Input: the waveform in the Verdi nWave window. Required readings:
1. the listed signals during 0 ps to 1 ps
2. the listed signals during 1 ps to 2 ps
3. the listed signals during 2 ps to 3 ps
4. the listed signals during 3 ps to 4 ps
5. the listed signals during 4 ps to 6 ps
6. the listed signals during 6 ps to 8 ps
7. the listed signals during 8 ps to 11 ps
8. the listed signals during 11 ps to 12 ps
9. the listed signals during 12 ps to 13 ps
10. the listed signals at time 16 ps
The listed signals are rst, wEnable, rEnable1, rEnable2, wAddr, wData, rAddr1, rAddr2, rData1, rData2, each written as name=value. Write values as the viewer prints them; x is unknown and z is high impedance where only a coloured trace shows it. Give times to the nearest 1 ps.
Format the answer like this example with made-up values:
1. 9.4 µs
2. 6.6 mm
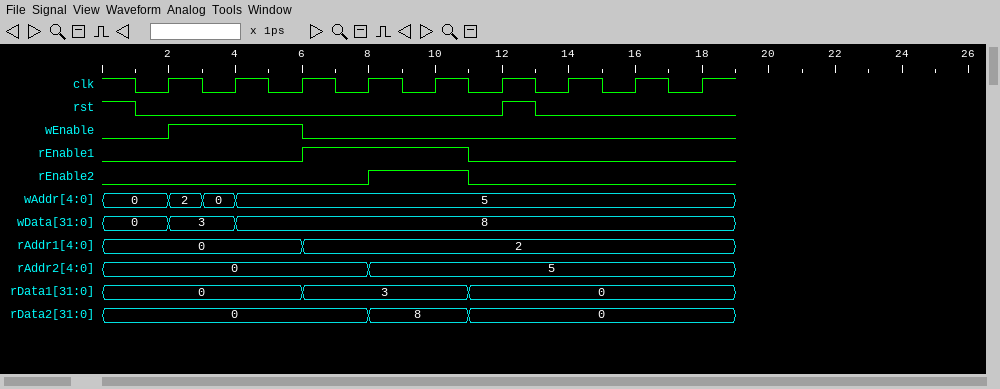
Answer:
1. rst=1, wEnable=0, rEnable1=0, rEnable2=0, wAddr=0, wData=0, rAddr1=0, rAddr2=0, rData1=0, rData2=0
2. rst=0, wEnable=0, rEnable1=0, rEnable2=0, wAddr=0, wData=0, rAddr1=0, rAddr2=0, rData1=0, rData2=0
3. rst=0, wEnable=1, rEnable1=0, rEnable2=0, wAddr=2, wData=3, rAddr1=0, rAddr2=0, rData1=0, rData2=0
4. rst=0, wEnable=1, rEnable1=0, rEnable2=0, wAddr=0, wData=3, rAddr1=0, rAddr2=0, rData1=0, rData2=0
5. rst=0, wEnable=1, rEnable1=0, rEnable2=0, wAddr=5, wData=8, rAddr1=0, rAddr2=0, rData1=0, rData2=0
6. rst=0, wEnable=0, rEnable1=1, rEnable2=0, wAddr=5, wData=8, rAddr1=2, rAddr2=0, rData1=3, rData2=0
7. rst=0, wEnable=0, rEnable1=1, rEnable2=1, wAddr=5, wData=8, rAddr1=2, rAddr2=5, rData1=3, rData2=8
8. rst=0, wEnable=0, rEnable1=0, rEnable2=0, wAddr=5, wData=8, rAddr1=2, rAddr2=5, rData1=0, rData2=0
9. rst=1, wEnable=0, rEnable1=0, rEnable2=0, wAddr=5, wData=8, rAddr1=2, rAddr2=5, rData1=0, rData2=0
10. rst=0, wEnable=0, rEnable1=0, rEnable2=0, wAddr=5, wData=8, rAddr1=2, rAddr2=5, rData1=0, rData2=0
